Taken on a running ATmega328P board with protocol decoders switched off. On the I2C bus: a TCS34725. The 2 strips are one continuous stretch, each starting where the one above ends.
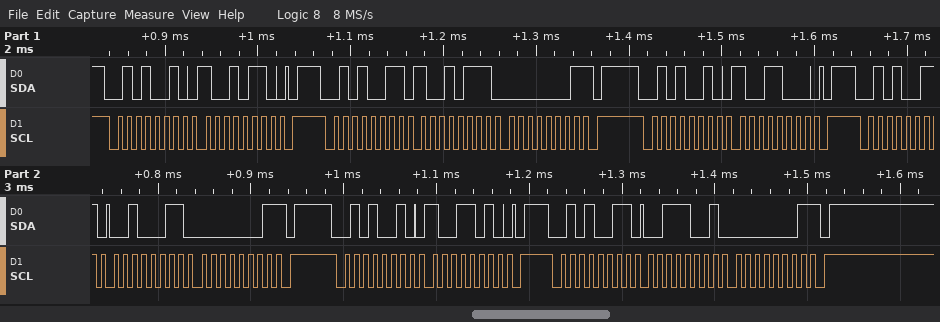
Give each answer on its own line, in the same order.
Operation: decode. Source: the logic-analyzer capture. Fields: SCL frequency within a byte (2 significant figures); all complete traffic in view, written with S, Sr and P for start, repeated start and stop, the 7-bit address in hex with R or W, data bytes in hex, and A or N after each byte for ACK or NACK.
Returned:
100 kHz
S 29W A 96 A P S 29R A 97 A 01 N P S 29W A 98 A P S 29R A 23 A 01 N P S 29W A 9A A P S 29R A 39 A 01 N P
